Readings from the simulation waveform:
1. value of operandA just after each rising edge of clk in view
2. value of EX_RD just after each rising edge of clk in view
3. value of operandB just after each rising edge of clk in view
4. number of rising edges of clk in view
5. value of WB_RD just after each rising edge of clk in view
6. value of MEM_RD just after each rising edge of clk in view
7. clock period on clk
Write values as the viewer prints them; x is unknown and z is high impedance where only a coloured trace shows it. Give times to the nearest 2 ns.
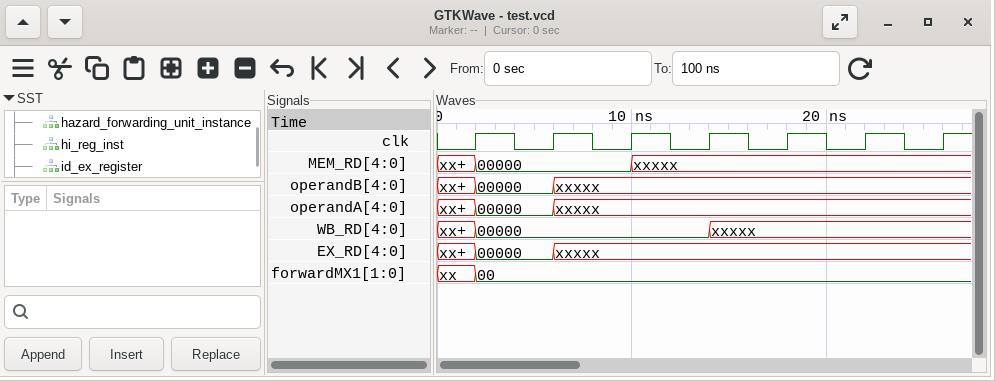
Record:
00000, xxxxx, xxxxx, xxxxx, xxxxx, xxxxx, xxxxx
00000, xxxxx, xxxxx, xxxxx, xxxxx, xxxxx, xxxxx
00000, xxxxx, xxxxx, xxxxx, xxxxx, xxxxx, xxxxx
7
00000, 00000, 00000, xxxxx, xxxxx, xxxxx, xxxxx
00000, 00000, xxxxx, xxxxx, xxxxx, xxxxx, xxxxx
4 ns
